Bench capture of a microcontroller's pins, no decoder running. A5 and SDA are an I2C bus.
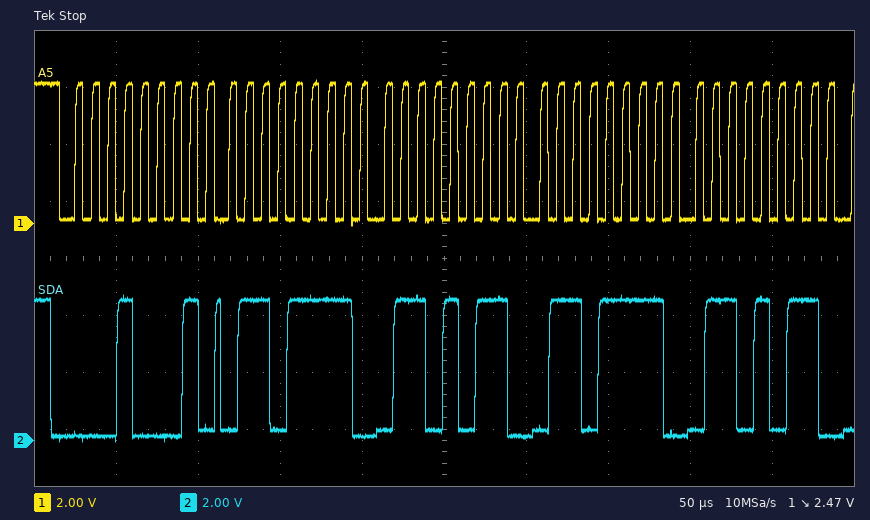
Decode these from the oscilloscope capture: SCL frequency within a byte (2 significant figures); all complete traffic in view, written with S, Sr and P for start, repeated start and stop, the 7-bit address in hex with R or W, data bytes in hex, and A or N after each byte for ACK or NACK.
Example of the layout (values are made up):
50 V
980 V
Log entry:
100 kHz
S 08R A 6F A 6B A 6F A 6B A
